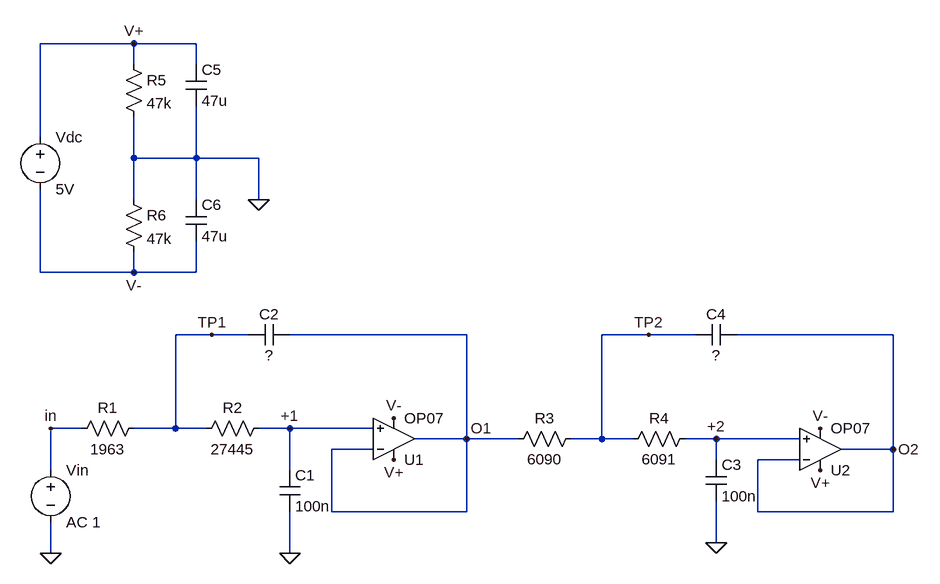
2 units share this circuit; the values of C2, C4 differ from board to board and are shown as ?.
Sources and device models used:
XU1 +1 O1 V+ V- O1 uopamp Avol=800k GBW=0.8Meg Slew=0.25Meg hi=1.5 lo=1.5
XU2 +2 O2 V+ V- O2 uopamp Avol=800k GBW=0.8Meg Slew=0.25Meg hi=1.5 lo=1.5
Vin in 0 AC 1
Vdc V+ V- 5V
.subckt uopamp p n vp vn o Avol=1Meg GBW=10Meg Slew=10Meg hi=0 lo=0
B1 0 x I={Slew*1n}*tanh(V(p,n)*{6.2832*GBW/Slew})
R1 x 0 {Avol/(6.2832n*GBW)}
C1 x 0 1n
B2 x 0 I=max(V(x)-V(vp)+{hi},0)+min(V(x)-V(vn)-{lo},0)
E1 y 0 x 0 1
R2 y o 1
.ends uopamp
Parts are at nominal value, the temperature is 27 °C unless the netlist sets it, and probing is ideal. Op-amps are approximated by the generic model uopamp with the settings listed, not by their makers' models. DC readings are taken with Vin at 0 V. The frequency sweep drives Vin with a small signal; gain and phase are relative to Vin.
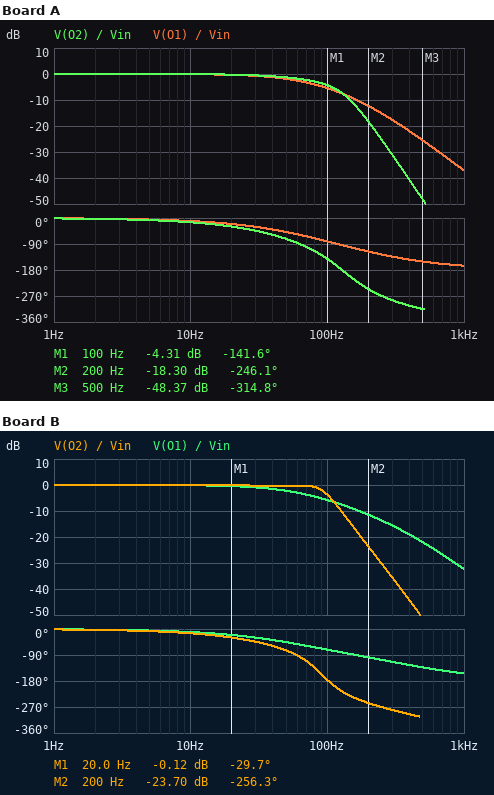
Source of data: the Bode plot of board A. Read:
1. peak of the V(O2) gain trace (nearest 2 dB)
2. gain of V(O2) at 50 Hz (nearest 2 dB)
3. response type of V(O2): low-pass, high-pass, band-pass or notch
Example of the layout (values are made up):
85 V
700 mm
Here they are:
0 dB
-2 dB
low-pass
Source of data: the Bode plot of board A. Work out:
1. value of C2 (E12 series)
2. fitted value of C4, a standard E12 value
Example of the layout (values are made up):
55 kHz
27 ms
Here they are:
330 nF
390 nF
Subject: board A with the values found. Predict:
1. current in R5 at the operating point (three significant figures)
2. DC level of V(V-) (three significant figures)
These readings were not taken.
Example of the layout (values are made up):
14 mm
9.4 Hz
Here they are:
53.2 µA
-2.50 V
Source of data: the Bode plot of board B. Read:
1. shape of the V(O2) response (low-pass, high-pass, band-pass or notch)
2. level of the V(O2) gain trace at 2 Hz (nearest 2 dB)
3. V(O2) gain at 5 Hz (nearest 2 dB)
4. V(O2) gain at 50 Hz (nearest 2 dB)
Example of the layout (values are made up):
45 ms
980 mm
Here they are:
low-pass
0 dB
0 dB
0 dB
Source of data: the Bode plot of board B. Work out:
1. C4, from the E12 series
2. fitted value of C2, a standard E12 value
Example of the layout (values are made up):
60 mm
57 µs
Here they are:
820 nF
180 nF
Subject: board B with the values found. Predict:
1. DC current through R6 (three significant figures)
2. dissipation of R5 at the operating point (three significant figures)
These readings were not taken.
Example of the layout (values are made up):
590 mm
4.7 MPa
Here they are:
53.2 µA
133 µW
